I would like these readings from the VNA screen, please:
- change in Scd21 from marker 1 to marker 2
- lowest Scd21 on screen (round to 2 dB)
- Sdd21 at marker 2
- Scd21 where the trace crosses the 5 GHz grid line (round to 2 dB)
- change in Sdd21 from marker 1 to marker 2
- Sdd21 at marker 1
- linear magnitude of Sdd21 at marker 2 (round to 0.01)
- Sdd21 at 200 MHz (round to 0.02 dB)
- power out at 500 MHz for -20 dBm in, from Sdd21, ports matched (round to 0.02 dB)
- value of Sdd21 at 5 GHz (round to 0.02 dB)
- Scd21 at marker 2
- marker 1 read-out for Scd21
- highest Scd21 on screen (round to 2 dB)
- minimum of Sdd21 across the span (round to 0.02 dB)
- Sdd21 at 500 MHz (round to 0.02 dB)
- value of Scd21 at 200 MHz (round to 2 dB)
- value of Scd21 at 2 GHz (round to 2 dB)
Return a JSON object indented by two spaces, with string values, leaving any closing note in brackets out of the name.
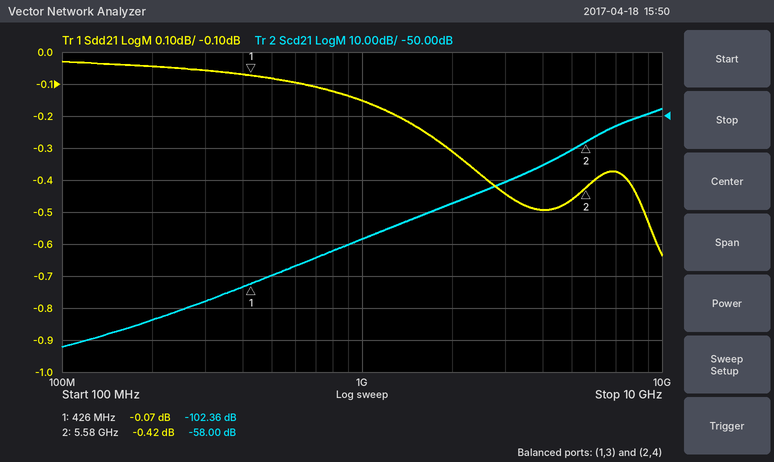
{
  "change in Scd21 from marker 1 to marker 2": "44.36 dB",
  "lowest Scd21 on screen": "-122 dB",
  "Sdd21 at marker 2": "-0.42 dB",
  "Scd21 where the trace crosses the 5 GHz grid line": "-60 dB",
  "change in Sdd21 from marker 1 to marker 2": "-0.35 dB",
  "Sdd21 at marker 1": "-0.07 dB",
  "linear magnitude of Sdd21 at marker 2": "0.95",
  "Sdd21 at 200 MHz": "-0.04 dB",
  "power out at 500 MHz for -20 dBm in, from Sdd21, ports matched": "-20.08 dBm",
  "value of Sdd21 at 5 GHz": "-0.46 dB",
  "Scd21 at marker 2": "-58.00 dB",
  "marker 1 read-out for Scd21": "-102.36 dB",
  "highest Scd21 on screen": "-48 dB",
  "minimum of Sdd21 across the span": "-0.64 dB",
  "Sdd21 at 500 MHz": "-0.08 dB",
  "value of Scd21 at 200 MHz": "-114 dB",
  "value of Scd21 at 2 GHz": "-78 dB"
}
